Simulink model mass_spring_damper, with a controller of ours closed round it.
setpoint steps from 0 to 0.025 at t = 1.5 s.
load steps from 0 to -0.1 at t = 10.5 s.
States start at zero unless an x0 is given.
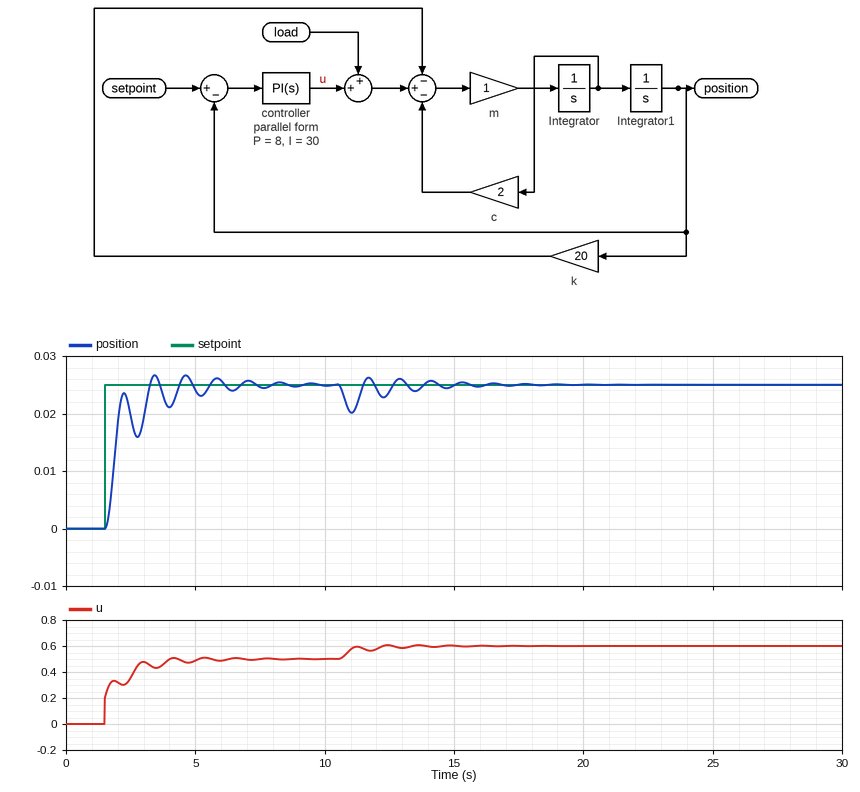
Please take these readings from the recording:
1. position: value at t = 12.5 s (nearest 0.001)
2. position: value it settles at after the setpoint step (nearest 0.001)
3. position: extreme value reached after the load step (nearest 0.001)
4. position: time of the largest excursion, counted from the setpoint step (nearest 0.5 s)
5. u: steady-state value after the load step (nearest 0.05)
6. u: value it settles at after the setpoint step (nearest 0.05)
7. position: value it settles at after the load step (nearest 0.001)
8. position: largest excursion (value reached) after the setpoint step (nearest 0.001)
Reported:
0.024
0.025
0.020
2.0 s
0.60
0.50
0.025
0.027
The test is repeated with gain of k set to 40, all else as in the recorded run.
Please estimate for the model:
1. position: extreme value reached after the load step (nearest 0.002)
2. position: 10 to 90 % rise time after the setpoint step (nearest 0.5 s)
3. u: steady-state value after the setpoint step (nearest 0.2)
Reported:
0.022
3.0 s
1.0
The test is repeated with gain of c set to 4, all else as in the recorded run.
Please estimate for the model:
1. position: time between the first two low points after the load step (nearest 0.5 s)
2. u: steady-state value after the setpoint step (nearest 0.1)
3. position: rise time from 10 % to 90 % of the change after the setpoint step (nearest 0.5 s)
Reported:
1.5 s
0.5
1.5 s
